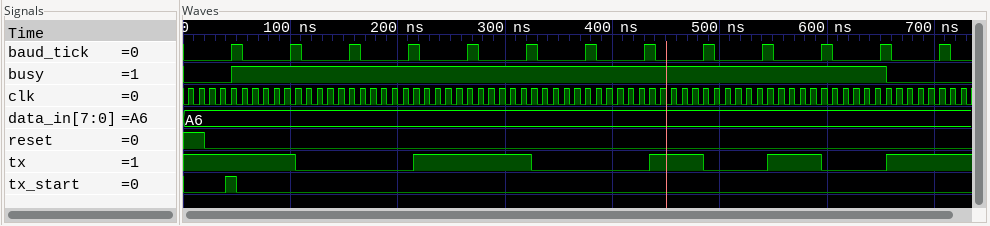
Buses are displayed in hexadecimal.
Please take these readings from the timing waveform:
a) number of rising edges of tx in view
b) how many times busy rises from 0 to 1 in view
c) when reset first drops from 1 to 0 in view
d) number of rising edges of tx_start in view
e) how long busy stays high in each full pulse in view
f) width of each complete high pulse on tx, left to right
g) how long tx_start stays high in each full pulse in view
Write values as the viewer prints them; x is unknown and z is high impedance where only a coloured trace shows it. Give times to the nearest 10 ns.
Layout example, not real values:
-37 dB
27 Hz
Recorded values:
4
1
20 ns
1
610 ns
110 ns, 50 ns, 50 ns
10 ns
